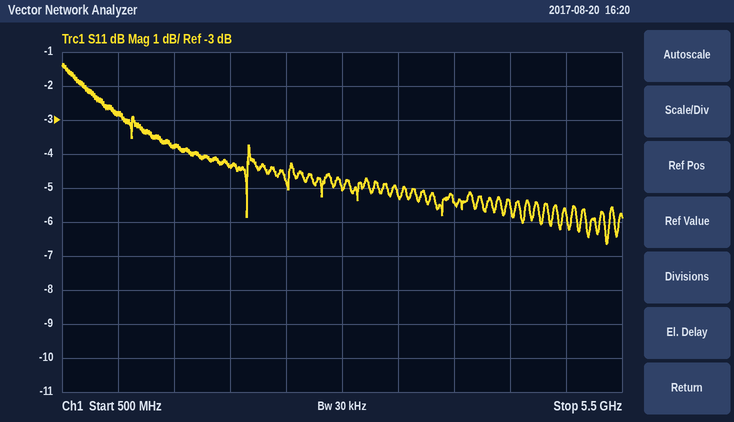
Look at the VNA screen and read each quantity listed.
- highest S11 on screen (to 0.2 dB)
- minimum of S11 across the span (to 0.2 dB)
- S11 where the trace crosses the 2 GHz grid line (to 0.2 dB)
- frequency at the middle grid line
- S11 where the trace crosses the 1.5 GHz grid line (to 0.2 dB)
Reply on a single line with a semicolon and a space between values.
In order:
-1.4 dB; -6.6 dB; -4.4 dB; 3 GHz; -3.8 dB
